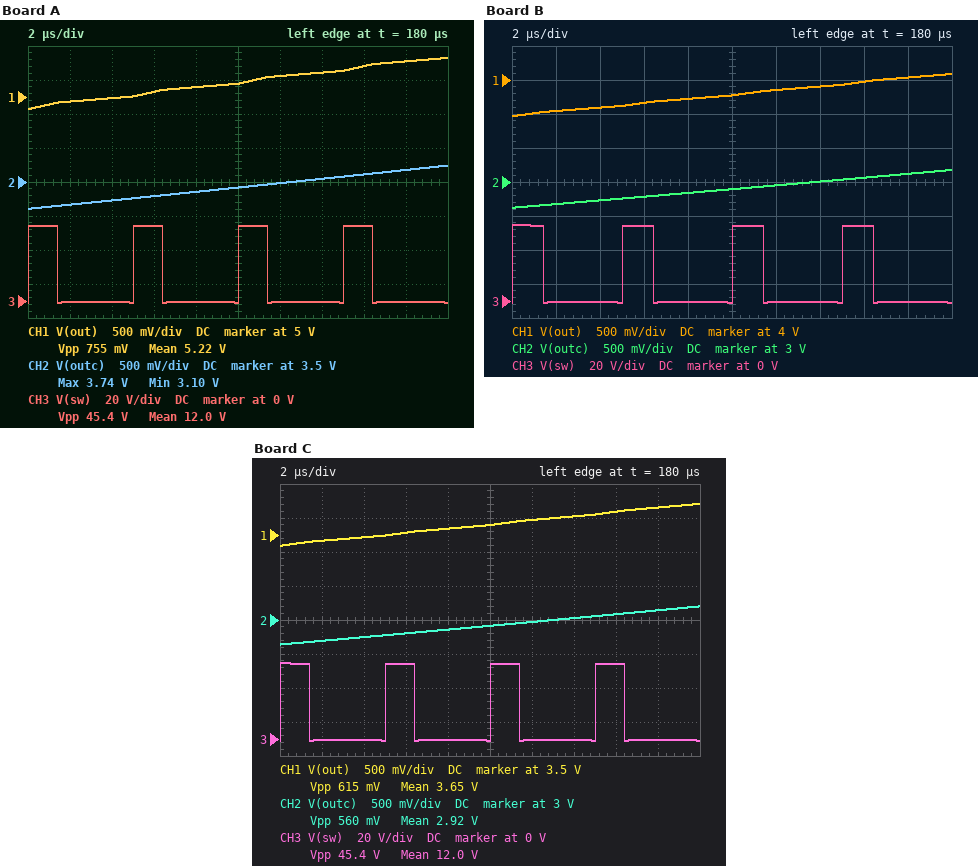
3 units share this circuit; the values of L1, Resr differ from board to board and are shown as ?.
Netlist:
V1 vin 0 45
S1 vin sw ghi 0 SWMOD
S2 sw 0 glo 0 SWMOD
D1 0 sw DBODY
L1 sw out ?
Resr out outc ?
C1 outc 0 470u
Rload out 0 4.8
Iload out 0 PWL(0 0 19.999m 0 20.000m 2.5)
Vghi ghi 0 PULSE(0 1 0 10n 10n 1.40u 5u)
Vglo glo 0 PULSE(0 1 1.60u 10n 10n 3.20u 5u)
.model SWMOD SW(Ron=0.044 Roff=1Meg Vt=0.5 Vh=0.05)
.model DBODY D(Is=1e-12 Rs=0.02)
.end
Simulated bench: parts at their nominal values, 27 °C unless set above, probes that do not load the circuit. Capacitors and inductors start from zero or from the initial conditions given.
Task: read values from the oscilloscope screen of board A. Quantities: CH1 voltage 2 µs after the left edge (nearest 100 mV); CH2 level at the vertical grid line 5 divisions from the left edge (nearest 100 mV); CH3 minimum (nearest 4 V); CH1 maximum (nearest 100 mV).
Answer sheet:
4.9 V
3.4 V
0 V
5.6 V
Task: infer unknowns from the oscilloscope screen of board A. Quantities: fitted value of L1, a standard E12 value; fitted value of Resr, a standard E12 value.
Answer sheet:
120 µH
0.12 Ω
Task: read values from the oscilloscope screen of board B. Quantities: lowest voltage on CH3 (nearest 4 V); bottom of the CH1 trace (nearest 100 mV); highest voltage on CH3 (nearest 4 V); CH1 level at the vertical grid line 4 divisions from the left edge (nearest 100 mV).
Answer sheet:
0 V
3.5 V
44 V
3.7 V
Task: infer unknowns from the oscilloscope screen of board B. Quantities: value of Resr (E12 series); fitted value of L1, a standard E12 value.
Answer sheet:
0.068 Ω
150 µH
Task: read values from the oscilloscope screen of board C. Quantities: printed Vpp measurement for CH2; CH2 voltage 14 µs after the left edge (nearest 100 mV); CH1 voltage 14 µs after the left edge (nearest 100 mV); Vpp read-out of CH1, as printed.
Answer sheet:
560 mV
3.0 V
3.8 V
615 mV
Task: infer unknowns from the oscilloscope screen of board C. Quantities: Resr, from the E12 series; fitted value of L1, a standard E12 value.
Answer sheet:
0.056 Ω
150 µH
